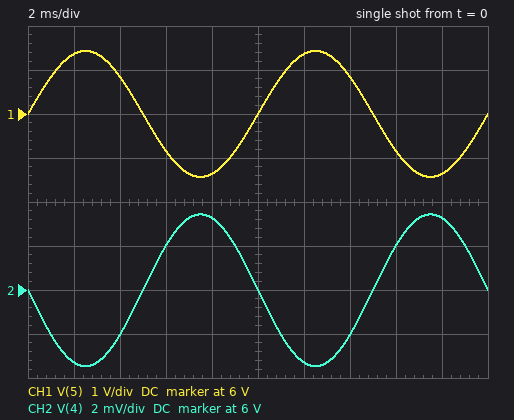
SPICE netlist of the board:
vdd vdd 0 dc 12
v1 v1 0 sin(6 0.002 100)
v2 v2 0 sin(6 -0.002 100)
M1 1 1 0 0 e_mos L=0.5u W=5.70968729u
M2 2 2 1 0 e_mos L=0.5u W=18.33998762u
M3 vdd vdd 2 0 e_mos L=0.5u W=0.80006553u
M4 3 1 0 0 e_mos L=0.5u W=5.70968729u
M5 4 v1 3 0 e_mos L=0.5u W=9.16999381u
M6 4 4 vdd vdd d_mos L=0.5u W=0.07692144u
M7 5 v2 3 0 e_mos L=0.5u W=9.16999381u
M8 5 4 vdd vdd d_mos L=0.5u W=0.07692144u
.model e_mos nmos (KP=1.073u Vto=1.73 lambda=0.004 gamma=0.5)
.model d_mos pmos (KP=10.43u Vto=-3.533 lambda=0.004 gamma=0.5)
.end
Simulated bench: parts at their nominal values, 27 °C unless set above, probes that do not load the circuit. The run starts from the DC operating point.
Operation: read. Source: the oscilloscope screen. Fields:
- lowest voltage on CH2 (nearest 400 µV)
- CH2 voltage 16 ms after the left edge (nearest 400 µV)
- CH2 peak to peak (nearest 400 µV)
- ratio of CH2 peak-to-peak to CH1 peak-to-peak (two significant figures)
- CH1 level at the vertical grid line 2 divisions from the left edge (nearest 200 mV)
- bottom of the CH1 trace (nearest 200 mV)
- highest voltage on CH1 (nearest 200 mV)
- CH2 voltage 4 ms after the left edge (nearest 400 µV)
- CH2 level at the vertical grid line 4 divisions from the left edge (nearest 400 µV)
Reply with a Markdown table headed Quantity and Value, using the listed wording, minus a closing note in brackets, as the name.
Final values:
| Quantity | Value |
|---|---|
| lowest voltage on CH2 | 5.9964 V |
| CH2 voltage 16 ms after the left edge | 6.0020 V |
| CH2 peak to peak | 6.8 mV |
| ratio of CH2 peak-to-peak to CH1 peak-to-peak | 0.0024 |
| CH1 level at the vertical grid line 2 divisions from the left edge | 6.8 V |
| bottom of the CH1 trace | 4.6 V |
| highest voltage on CH1 | 7.4 V |
| CH2 voltage 4 ms after the left edge | 5.9980 V |
| CH2 level at the vertical grid line 4 divisions from the left edge | 6.0032 V |
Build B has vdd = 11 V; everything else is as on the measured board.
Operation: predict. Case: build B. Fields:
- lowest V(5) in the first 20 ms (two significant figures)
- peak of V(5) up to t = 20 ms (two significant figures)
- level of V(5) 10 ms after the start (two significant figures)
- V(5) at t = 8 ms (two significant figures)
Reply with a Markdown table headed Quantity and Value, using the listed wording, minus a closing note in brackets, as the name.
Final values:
| Quantity | Value |
|---|---|
| lowest V(5) in the first 20 ms | 3.7 V |
| peak of V(5) up to t = 20 ms | 7.2 V |
| level of V(5) 10 ms after the start | 5.4 V |
| V(5) at t = 8 ms | 3.8 V |
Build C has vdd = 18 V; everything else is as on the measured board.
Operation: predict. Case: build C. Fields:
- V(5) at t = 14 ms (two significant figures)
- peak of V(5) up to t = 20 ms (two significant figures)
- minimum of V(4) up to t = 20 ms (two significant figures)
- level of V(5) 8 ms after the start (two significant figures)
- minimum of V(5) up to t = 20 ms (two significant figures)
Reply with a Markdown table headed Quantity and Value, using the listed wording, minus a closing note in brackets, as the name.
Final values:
| Quantity | Value |
|---|---|
| V(5) at t = 14 ms | 9.9 V |
| peak of V(5) up to t = 20 ms | 10 V |
| minimum of V(4) up to t = 20 ms | 9.4 V |
| level of V(5) 8 ms after the start | 8.8 V |
| minimum of V(5) up to t = 20 ms | 8.7 V |
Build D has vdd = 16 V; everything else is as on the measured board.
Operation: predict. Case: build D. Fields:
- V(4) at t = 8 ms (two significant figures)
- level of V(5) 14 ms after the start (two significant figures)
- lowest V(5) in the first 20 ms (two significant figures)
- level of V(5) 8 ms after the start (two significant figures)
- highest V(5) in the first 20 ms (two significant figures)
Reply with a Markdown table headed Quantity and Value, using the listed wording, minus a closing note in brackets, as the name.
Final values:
| Quantity | Value |
|---|---|
| V(4) at t = 8 ms | 8.3 V |
| level of V(5) 14 ms after the start | 8.8 V |
| lowest V(5) in the first 20 ms | 7.4 V |
| level of V(5) 8 ms after the start | 7.5 V |
| highest V(5) in the first 20 ms | 9.1 V |
